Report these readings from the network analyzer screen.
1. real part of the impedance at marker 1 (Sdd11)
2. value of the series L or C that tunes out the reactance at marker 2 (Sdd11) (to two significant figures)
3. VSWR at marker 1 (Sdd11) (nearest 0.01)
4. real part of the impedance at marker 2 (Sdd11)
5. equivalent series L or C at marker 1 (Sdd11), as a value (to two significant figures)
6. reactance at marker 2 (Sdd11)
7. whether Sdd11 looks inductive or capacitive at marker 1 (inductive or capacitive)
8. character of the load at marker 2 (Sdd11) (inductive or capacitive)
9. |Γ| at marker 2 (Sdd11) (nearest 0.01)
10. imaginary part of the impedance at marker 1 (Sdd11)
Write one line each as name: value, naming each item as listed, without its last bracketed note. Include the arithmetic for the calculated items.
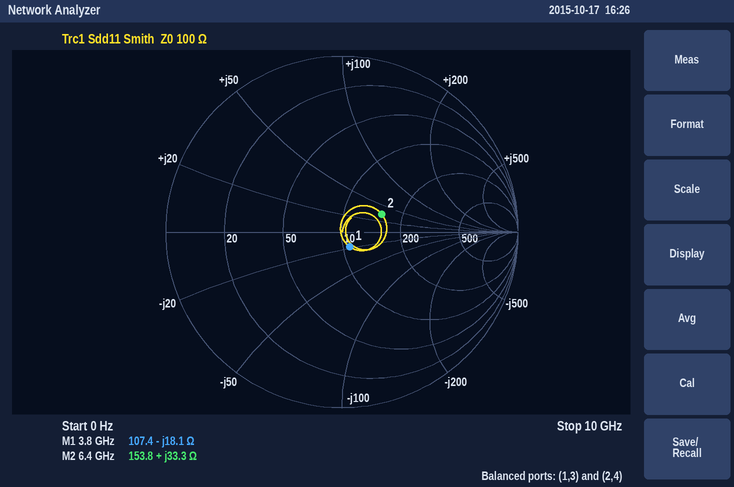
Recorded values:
real part of the impedance at marker 1: 107.4 Ω
value of the series L or C that tunes out the reactance at marker 2 (Sdd11): C = 1/(2π × 6.4 GHz × 33.3 Ω) ≈ 747 fF, so 750 fF to two significant figures
VSWR at marker 1 (Sdd11): 1.21
real part of the impedance at marker 2: 153.8 Ω
equivalent series L or C at marker 1 (Sdd11), as a value: C = 1/(2π × 3.8 GHz × 18.1 Ω) ≈ 2.3 pF
reactance at marker 2: +33.3 Ω
whether Sdd11 looks inductive or capacitive at marker 1: capacitive
character of the load at marker 2 (Sdd11): inductive
|Γ| at marker 2 (Sdd11): 0.25
imaginary part of the impedance at marker 1: -18.1 Ω
